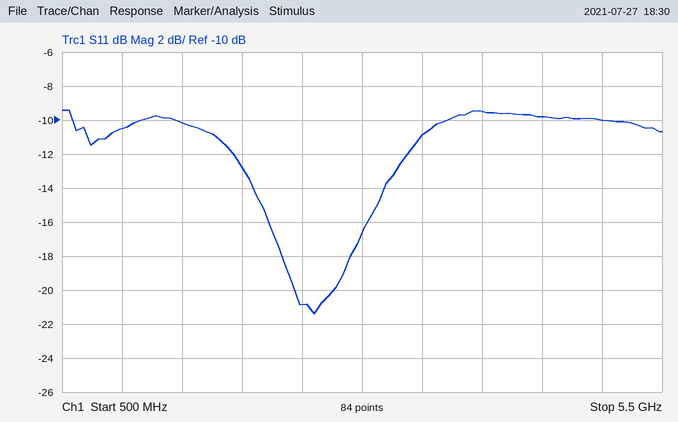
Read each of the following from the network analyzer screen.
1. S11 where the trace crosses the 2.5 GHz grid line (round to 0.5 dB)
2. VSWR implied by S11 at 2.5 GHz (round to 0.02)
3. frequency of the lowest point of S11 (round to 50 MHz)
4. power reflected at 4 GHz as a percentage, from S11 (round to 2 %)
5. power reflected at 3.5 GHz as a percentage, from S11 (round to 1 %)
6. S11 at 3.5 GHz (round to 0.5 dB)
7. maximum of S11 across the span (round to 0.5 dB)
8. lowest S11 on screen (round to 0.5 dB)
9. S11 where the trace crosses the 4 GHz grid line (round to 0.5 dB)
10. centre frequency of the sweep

-21.0 dB
1.20
2.60 GHz
12 %
8 %
-11.0 dB
-9.5 dB
-21.5 dB
-9.5 dB
3 GHz
